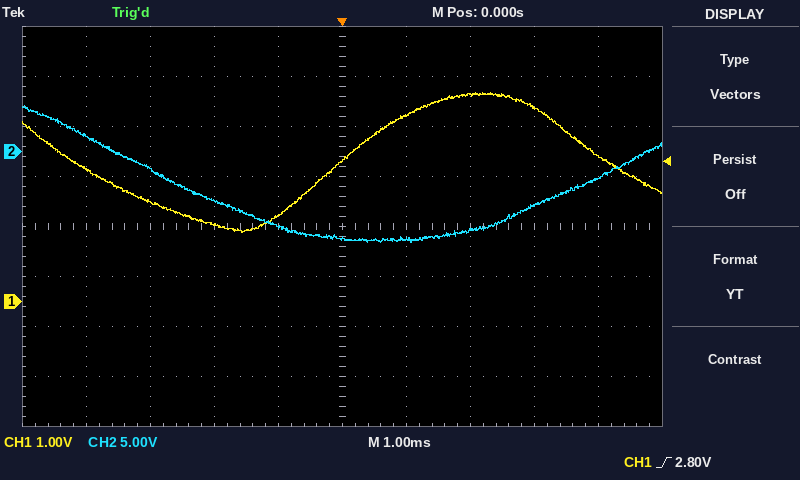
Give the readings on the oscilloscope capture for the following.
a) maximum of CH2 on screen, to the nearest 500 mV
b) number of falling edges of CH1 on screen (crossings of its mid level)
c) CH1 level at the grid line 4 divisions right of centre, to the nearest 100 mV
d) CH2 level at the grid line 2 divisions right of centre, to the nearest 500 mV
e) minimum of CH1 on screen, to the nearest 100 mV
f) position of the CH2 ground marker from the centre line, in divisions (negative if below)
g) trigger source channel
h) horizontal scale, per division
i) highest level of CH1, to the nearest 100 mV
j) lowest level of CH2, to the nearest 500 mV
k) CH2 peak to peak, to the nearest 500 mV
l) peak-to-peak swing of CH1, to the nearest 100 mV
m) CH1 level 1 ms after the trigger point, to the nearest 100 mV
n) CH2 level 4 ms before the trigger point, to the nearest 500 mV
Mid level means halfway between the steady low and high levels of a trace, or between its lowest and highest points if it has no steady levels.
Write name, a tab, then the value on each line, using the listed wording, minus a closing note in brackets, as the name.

maximum of CH2 on screen, to the nearest 500 mV	4.5 V
number of falling edges of CH1 on screen	2
CH1 level at the grid line 4 divisions right of centre, to the nearest 100 mV	2.9 V
CH2 level at the grid line 2 divisions right of centre, to the nearest 500 mV	-8.0 V
minimum of CH1 on screen, to the nearest 100 mV	1.4 V
position of the CH2 ground marker from the centre line, in divisions	+1.5 div
trigger source channel	CH1
horizontal scale, per division	1 ms
highest level of CH1, to the nearest 100 mV	4.2 V
lowest level of CH2, to the nearest 500 mV	-9.0 V
CH2 peak to peak, to the nearest 500 mV	13.5 V
peak-to-peak swing of CH1, to the nearest 100 mV	2.8 V
CH1 level 1 ms after the trigger point, to the nearest 100 mV	3.7 V
CH2 level 4 ms before the trigger point, to the nearest 500 mV	1.5 V
